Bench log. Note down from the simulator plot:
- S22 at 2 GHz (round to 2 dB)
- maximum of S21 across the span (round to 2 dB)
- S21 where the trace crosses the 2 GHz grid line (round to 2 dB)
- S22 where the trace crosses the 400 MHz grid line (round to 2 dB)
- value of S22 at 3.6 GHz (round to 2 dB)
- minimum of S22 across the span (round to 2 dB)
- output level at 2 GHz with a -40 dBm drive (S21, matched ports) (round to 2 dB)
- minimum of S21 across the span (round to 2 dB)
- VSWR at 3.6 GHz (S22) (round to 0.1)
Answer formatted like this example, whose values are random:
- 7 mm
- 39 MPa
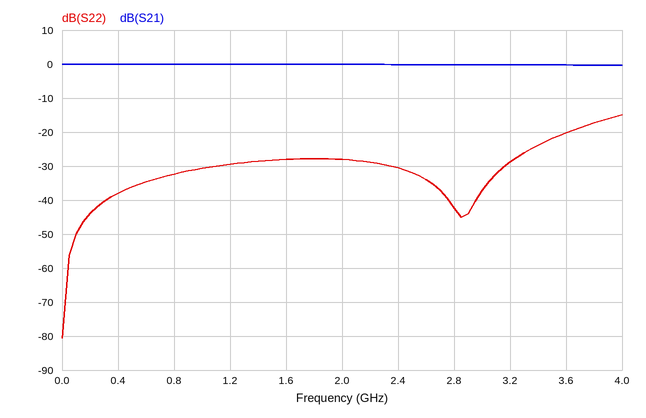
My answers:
- -28 dB
- 0 dB
- 0 dB
- -38 dB
- -20 dB
- -80 dB
- -40 dBm
- 0 dB
- 1.2
